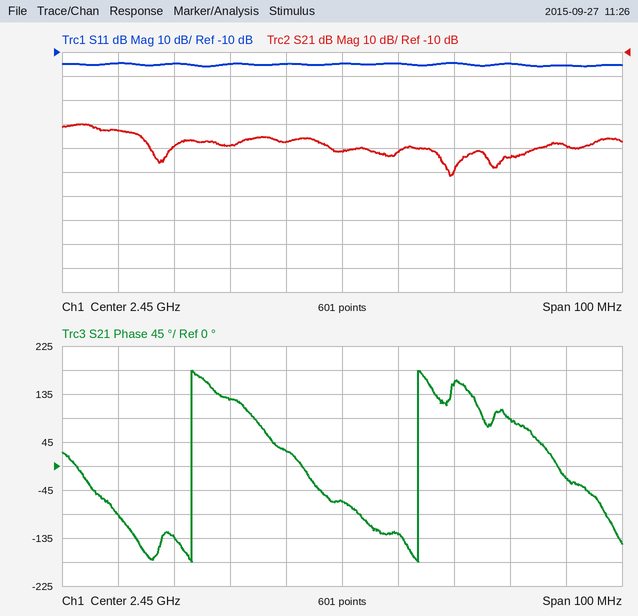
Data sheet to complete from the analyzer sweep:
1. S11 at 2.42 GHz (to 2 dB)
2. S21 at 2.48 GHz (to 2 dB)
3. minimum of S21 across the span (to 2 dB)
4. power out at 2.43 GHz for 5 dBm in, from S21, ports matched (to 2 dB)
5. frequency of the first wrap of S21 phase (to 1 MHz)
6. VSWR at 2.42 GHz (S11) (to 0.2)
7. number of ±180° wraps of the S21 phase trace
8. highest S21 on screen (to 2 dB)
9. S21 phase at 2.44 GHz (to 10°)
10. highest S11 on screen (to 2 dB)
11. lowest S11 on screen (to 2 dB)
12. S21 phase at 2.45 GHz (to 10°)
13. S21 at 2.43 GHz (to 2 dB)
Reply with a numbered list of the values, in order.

1. -14 dB
2. -54 dB
3. -62 dB
4. -44 dBm
5. 2.423 GHz
6. 1.4
7. 2
8. -40 dB
9. 30°
10. -14 dB
11. -16 dB
12. -70°
13. -48 dB
